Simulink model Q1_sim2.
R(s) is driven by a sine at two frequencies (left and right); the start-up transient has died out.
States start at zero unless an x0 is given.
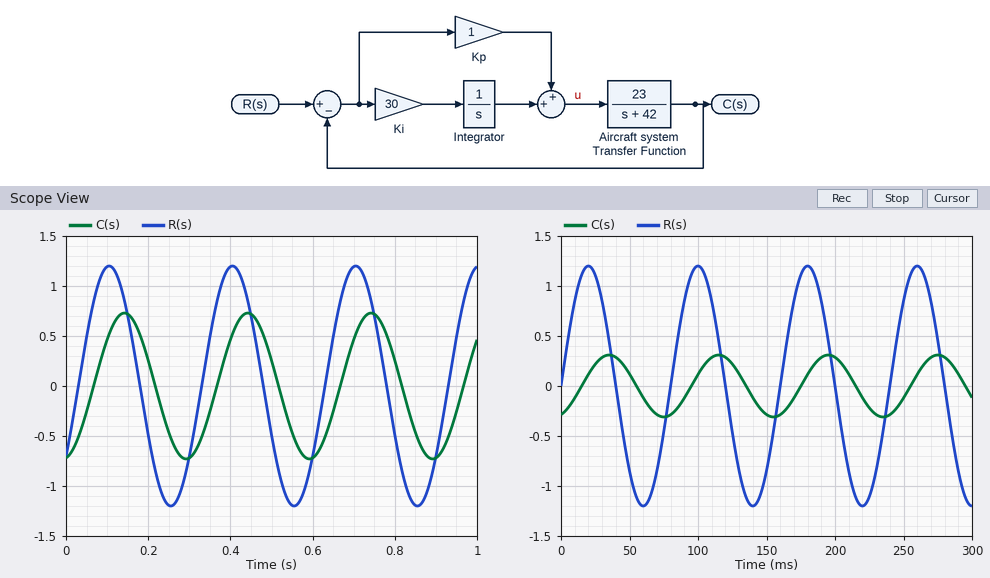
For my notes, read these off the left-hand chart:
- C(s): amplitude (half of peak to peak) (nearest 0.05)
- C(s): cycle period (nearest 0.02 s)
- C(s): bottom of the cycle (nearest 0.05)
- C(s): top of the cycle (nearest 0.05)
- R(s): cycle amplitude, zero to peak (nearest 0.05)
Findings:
0.75
0.30 s
-0.75
0.75
1.20
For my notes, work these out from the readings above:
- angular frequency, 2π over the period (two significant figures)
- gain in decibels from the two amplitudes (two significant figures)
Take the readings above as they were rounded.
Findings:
21 rad/s
-4.1 dB
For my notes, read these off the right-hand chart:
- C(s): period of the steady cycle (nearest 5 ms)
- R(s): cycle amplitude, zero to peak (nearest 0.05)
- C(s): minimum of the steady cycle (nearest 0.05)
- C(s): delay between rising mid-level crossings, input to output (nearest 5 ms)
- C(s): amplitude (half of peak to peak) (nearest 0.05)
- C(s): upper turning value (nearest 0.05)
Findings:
80 ms
1.20
-0.30
15 ms
0.30
0.30
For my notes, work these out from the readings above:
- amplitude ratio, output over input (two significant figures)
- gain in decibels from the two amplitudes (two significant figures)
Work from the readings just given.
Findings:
0.25
-12 dB
